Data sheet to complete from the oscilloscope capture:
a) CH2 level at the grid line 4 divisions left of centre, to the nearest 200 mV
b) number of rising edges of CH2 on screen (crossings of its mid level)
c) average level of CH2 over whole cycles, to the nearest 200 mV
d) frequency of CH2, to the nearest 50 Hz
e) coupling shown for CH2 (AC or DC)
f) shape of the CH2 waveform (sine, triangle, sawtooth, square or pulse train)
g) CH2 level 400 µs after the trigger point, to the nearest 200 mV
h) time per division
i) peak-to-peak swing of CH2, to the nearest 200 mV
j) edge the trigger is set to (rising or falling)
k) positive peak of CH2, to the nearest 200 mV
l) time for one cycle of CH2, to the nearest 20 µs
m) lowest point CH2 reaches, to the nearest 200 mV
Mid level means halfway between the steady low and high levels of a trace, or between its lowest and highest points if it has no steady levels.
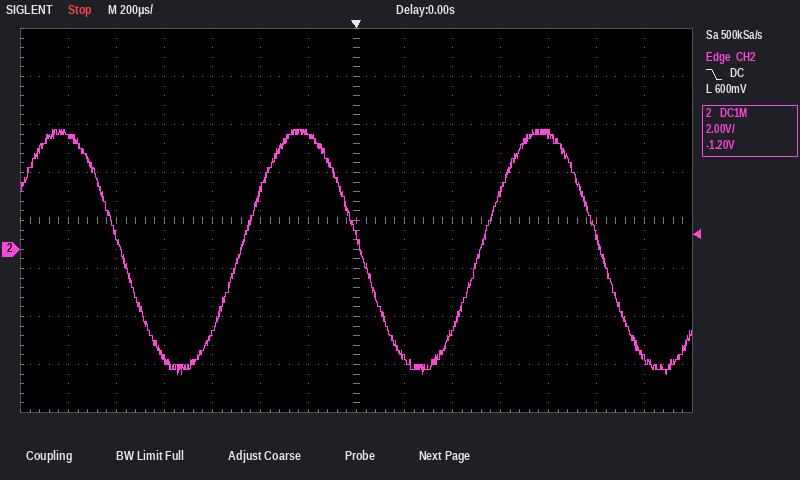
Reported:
-4.6 V
2
0.0 V
1.00 kHz
DC
sine
-3.4 V
200 µs
10.2 V
falling
5.0 V
1.00 ms
-5.2 V
